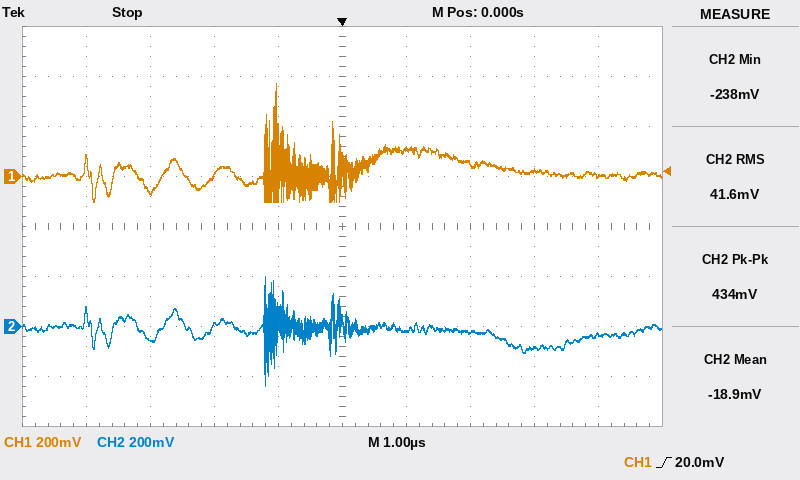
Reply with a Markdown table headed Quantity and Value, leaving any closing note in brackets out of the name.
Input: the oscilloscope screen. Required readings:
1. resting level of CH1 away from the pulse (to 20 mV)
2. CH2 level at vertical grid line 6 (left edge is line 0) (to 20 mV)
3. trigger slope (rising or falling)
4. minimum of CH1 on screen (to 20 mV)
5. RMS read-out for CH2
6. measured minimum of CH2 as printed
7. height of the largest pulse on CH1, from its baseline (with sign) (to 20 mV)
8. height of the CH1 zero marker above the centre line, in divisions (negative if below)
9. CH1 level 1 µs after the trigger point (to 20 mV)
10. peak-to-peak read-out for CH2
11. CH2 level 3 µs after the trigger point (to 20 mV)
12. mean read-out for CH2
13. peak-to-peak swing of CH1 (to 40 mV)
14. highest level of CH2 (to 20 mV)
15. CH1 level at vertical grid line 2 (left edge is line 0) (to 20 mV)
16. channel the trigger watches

| Quantity | Value |
|---|---|
| resting level of CH1 away from the pulse | 0 mV |
| CH2 level at vertical grid line 6 (left edge is line 0) | -20 mV |
| trigger slope | rising |
| minimum of CH1 on screen | -100 mV |
| RMS read-out for CH2 | 41.6 mV |
| measured minimum of CH2 as printed | -238 mV |
| height of the largest pulse on CH1, from its baseline (with sign) | +360 mV |
| height of the CH1 zero marker above the centre line, in divisions | +1.0 div |
| CH1 level 1 µs after the trigger point | 100 mV |
| peak-to-peak read-out for CH2 | 434 mV |
| CH2 level 3 µs after the trigger point | -80 mV |
| mean read-out for CH2 | -18.9 mV |
| peak-to-peak swing of CH1 | 480 mV |
| highest level of CH2 | 200 mV |
| CH1 level at vertical grid line 2 (left edge is line 0) | -60 mV |
| channel the trigger watches | CH1 |
